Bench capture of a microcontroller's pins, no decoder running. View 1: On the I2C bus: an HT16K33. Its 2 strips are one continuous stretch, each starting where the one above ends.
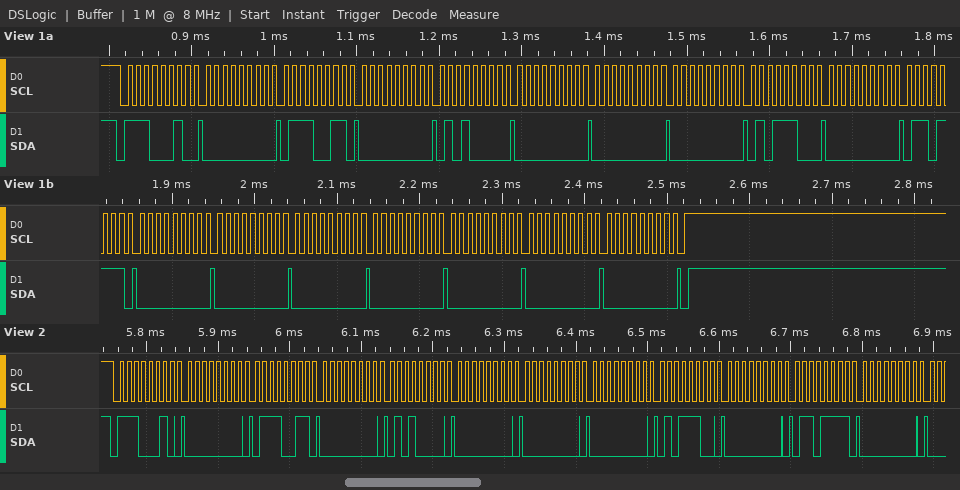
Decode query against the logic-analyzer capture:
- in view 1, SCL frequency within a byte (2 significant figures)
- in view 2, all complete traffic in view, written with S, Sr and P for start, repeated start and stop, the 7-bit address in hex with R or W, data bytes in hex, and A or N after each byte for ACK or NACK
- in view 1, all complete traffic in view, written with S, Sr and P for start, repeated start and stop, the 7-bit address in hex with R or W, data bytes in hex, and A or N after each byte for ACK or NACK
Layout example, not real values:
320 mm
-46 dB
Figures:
100 kHz
S 71W A 00 A 73 A 00 A 50 A 00 A 00 A 00 A 5C A 00 A 6F A 00 A
S 71W A 00 A 73 A 00 A 50 A 00 A 00 A 00 A 5C A 00 A 6F A 00 A 00 A 00 A 00 A 00 A 00 A 00 A P
